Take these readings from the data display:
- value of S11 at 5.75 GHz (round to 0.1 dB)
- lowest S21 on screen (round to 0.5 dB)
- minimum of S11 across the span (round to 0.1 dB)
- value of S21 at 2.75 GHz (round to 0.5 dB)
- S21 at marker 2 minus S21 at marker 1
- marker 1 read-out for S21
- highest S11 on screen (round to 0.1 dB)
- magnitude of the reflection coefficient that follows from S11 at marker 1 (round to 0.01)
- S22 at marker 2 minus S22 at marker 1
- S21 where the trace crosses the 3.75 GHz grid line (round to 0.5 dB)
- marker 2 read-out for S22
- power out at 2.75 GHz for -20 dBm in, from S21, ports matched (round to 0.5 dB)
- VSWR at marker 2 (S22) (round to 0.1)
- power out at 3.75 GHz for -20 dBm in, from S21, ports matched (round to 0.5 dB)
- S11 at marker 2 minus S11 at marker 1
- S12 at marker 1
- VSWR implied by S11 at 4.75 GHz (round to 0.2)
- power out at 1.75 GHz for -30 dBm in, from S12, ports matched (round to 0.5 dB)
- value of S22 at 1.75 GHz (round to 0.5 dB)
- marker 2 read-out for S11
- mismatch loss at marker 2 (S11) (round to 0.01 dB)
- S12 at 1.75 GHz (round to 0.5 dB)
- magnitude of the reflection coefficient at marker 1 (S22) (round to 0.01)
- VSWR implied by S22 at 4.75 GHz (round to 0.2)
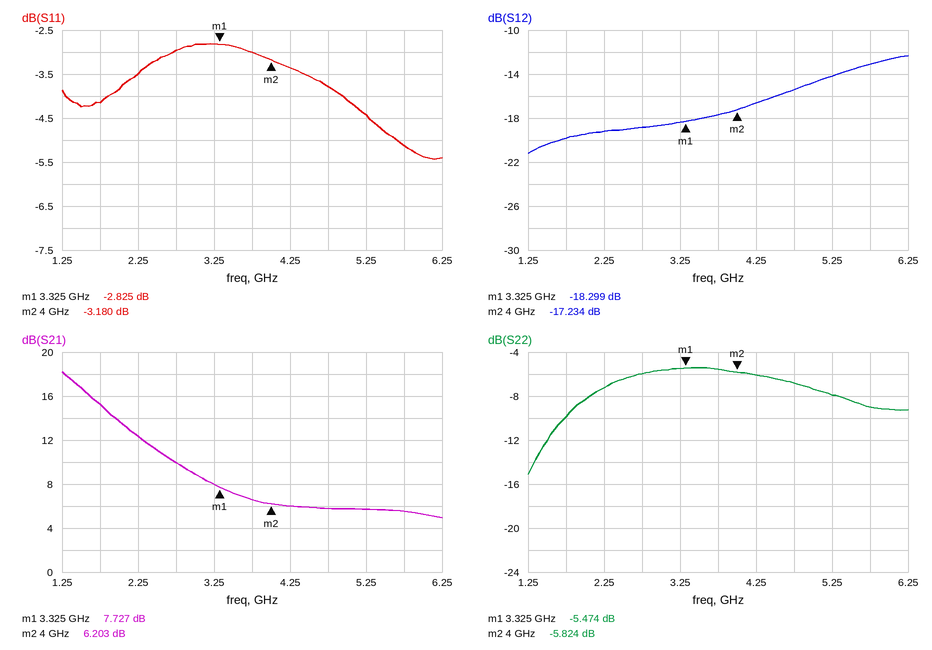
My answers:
-5.1 dB
5.0 dB
-5.4 dB
10.0 dB
-1.524 dB
7.727 dB
-2.8 dB
0.72
-0.350 dB
6.5 dB
-5.824 dB
-10.0 dBm
3.1
-13.5 dBm
-0.355 dB
-18.299 dB
4.6
-50.0 dBm
-10.0 dB
-3.180 dB
2.85 dB
-20.0 dB
0.53
2.6
